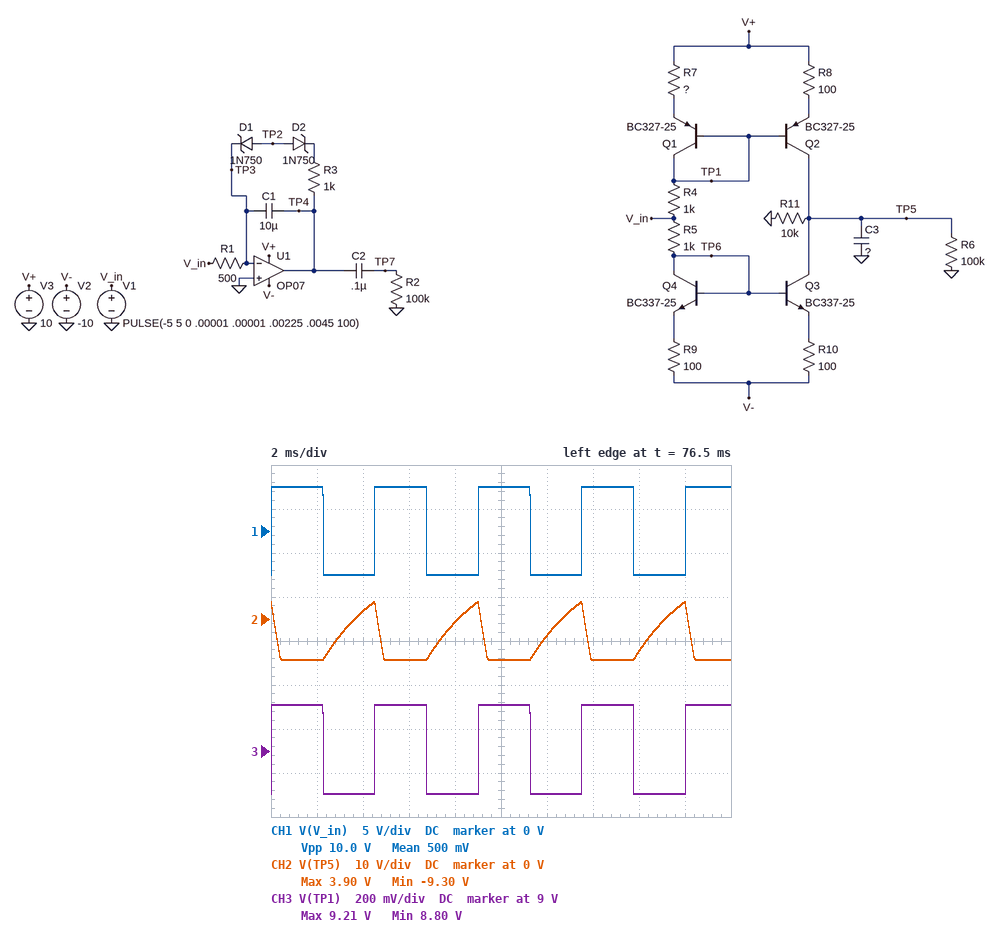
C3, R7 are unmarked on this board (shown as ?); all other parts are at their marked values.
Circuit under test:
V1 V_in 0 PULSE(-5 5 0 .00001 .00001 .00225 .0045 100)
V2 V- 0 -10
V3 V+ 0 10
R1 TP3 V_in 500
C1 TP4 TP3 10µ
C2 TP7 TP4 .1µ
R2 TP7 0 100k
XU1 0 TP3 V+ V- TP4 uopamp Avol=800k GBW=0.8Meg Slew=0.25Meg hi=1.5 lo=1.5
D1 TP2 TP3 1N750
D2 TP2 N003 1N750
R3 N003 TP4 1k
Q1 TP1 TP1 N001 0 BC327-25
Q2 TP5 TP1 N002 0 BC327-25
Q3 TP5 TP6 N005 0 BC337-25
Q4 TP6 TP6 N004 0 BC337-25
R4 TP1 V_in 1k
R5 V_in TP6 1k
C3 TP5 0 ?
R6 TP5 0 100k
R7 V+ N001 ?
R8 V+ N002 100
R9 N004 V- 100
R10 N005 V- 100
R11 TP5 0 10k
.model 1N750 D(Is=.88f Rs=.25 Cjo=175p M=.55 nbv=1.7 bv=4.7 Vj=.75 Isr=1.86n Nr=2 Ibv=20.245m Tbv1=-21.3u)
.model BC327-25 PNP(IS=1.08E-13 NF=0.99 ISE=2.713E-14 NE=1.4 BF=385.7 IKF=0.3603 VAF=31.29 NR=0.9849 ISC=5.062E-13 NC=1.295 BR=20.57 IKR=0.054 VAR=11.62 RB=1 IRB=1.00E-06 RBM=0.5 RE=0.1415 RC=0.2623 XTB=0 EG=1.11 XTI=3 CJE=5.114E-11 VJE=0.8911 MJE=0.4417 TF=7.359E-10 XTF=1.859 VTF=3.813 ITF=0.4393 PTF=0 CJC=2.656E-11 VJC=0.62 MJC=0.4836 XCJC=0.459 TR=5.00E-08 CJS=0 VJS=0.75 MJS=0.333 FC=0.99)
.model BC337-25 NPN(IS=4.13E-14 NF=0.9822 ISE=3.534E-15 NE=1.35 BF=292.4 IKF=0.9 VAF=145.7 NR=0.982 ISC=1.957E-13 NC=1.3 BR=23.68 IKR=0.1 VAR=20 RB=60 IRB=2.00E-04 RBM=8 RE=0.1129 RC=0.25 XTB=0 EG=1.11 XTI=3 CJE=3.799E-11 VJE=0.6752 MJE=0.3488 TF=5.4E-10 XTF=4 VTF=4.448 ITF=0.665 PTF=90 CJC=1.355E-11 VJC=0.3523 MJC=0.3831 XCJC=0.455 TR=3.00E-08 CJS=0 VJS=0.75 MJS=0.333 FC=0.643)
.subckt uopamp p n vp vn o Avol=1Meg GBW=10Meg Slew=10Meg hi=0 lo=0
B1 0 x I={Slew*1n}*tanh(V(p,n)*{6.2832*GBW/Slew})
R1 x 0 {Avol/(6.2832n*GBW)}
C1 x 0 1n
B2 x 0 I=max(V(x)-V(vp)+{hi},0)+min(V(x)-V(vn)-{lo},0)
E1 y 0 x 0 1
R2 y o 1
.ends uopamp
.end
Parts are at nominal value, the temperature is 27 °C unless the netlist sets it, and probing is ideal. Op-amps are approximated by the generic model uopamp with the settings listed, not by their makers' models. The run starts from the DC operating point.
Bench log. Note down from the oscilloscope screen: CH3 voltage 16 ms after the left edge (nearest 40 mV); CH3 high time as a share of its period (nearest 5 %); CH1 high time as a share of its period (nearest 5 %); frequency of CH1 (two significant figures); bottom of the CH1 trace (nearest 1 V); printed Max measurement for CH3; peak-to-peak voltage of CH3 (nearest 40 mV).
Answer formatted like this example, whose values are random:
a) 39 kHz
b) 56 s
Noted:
a) 8.80 V
b) 50 %
c) 50 %
d) 220 Hz
e) -5 V
f) 9.21 V
g) 400 mV
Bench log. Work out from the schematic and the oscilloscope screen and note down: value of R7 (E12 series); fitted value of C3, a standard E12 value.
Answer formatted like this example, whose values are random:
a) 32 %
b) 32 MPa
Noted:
a) 39 Ω
b) 330 nF
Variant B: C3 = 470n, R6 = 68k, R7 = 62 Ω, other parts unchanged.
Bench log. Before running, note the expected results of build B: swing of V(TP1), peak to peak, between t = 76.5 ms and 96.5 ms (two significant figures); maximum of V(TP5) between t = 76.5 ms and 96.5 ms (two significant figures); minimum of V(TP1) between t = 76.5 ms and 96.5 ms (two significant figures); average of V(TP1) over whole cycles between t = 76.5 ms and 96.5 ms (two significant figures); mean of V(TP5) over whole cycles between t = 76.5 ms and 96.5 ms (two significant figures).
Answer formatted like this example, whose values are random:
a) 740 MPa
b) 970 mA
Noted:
a) 610 mV
b) 9.3 V
c) 8.5 V
d) 8.8 V
e) -2.0 V
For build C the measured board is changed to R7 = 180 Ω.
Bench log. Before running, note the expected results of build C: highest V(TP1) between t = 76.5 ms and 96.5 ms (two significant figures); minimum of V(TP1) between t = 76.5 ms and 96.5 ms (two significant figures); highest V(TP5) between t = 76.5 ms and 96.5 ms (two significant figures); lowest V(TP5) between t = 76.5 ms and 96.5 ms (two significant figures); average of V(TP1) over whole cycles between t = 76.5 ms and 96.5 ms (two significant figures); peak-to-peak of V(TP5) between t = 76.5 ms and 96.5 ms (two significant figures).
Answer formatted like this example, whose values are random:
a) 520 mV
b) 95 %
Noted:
a) 8.7 V
b) 7.2 V
c) 8.9 V
d) -9.0 V
e) 8.4 V
f) 18 V
